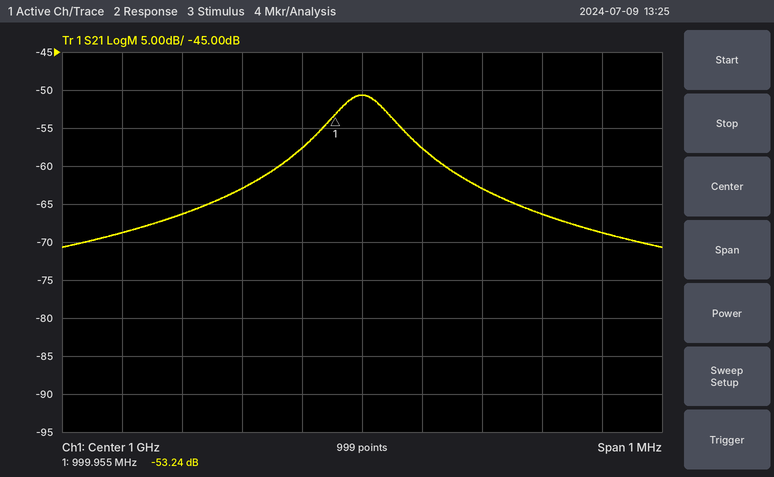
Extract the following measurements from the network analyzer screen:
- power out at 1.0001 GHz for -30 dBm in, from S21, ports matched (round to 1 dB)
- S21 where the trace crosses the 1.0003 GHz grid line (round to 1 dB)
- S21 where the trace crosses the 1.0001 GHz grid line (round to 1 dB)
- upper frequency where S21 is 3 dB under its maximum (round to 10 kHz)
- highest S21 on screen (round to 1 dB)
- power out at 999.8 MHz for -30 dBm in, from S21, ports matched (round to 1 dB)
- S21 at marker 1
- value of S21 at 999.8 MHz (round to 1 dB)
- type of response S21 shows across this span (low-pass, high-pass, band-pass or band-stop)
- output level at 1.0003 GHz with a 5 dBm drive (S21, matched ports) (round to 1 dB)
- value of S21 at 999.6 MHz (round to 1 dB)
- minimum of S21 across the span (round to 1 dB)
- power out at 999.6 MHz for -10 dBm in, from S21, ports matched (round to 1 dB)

-88 dBm
-66 dB
-58 dB
1.00005 GHz
-51 dB
-93 dBm
-53.24 dB
-63 dB
band-pass
-61 dBm
-69 dB
-71 dB
-79 dBm
